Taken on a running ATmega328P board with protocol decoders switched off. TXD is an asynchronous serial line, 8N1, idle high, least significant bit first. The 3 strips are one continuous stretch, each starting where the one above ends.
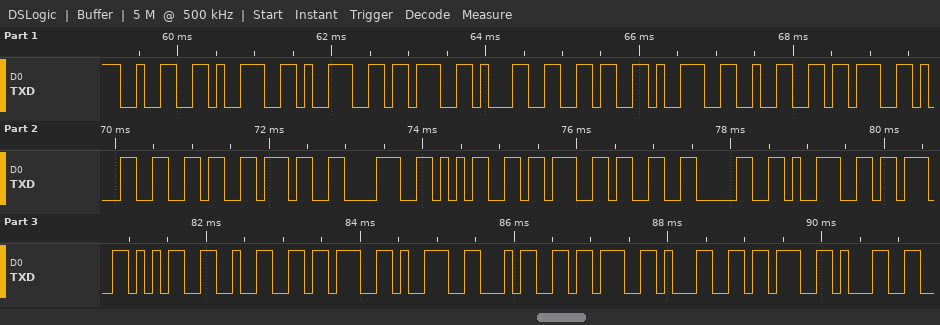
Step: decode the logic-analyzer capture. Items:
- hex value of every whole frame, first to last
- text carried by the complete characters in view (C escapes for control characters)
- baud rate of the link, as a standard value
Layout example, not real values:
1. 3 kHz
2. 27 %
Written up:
1. 32 39 39 3B 31 36 39 32 3B 31 36 37 38 35 3B 33 30 39 3B 35 32 3B 39 34 3B 31 3B 31
2. "299;1692;16785;309;52;94;1;1"
3. 9600 baud
